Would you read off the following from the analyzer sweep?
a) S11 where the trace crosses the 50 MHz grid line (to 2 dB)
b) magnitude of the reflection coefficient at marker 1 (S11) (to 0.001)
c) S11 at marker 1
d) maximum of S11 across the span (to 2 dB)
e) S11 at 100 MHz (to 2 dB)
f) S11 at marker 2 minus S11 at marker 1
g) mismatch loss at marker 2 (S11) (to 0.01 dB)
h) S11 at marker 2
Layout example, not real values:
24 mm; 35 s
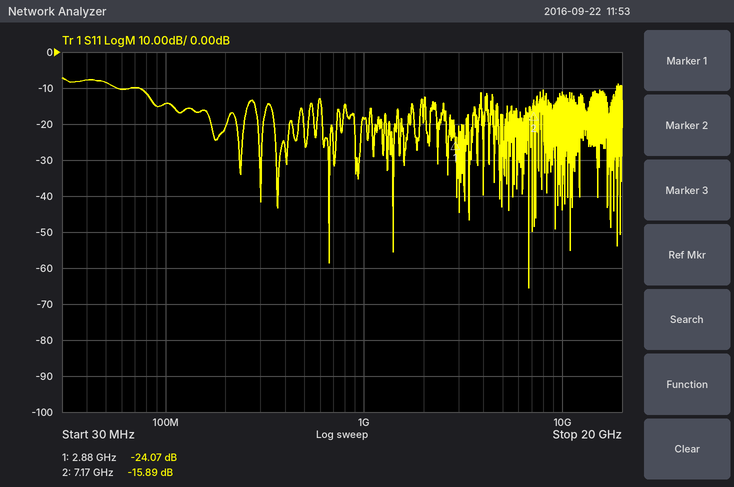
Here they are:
-8 dB; 0.063; -24.07 dB; -8 dB; -14 dB; 8.18 dB; 0.11 dB; -15.89 dB
